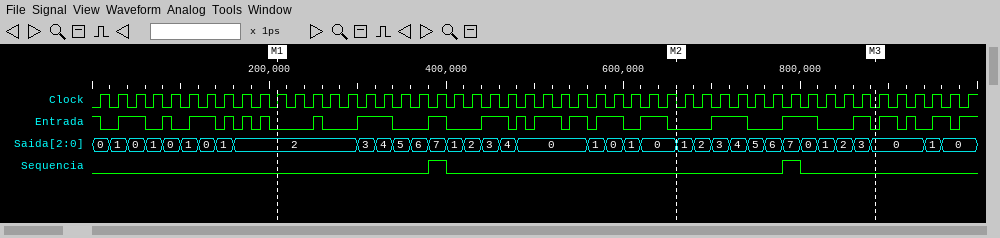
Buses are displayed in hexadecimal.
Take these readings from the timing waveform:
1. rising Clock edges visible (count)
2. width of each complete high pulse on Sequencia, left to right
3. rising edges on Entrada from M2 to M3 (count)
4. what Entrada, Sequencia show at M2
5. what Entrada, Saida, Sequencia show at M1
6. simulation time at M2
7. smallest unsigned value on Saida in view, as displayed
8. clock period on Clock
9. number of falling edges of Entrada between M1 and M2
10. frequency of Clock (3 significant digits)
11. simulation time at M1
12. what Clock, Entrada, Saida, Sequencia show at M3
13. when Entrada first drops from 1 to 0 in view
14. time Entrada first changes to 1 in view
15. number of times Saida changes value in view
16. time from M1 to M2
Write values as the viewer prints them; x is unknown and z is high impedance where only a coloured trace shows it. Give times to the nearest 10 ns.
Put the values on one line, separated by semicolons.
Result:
50; 20 ns, 20 ns; 3; Entrada=0, Sequencia=0; Entrada=0, Saida=2, Sequencia=0; 660 ns; 0; 20 ns; 9; 50.0 MHz; 210 ns; Clock=0, Entrada=0, Saida=0, Sequencia=0; 10 ns; 30 ns; 36; 450 ns
